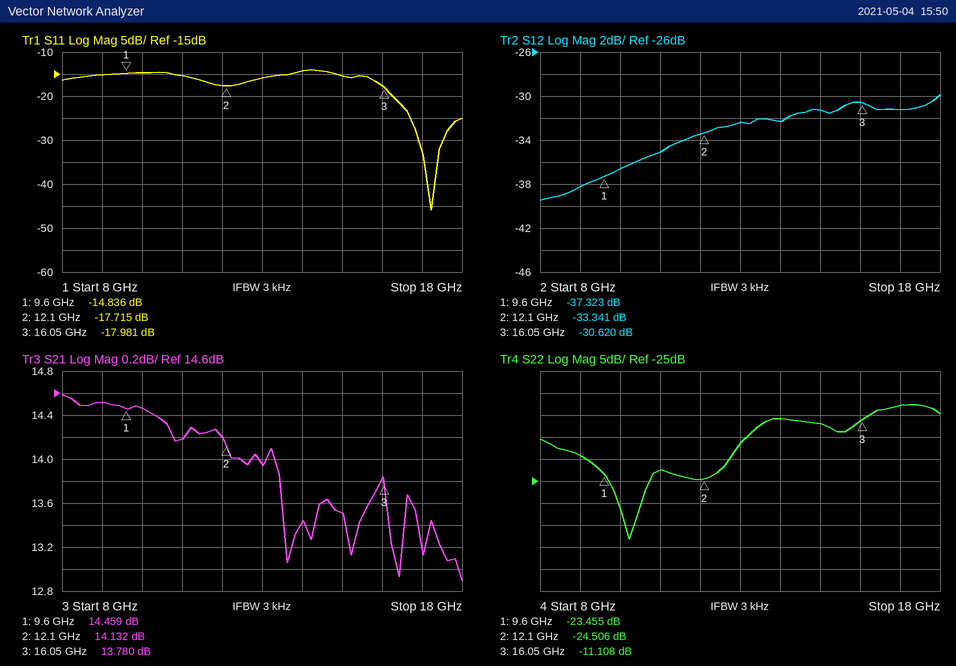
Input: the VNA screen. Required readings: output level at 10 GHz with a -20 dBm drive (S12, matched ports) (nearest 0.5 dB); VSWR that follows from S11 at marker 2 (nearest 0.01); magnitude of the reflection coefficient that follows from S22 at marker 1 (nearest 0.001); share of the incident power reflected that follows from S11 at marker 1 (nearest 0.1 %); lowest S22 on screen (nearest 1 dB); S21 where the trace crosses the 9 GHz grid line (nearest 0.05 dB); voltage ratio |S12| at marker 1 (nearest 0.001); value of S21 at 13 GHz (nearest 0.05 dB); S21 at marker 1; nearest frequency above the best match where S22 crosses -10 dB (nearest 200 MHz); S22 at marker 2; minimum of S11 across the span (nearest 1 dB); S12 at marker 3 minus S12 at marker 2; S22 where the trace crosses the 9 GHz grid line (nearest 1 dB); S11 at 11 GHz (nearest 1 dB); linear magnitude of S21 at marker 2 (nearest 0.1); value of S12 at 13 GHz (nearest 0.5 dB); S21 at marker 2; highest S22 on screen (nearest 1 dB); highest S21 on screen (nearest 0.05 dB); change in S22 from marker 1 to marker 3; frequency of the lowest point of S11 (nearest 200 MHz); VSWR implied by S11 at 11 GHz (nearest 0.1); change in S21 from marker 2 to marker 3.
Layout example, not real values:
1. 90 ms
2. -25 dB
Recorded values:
1. -56.5 dBm
2. 1.30
3. 0.067
4. 3.3 %
5. -38 dB
6. 14.50 dB
7. 0.014
8. 13.95 dB
9. 14.459 dB
10. 16.2 GHz
11. -24.506 dB
12. -46 dB
13. 2.721 dB
14. -19 dB
15. -15 dB
16. 5.1
17. -32.5 dB
18. 14.132 dB
19. -8 dB
20. 14.60 dB
21. 12.347 dB
22. 17.2 GHz
23. 1.4
24. -0.352 dB
